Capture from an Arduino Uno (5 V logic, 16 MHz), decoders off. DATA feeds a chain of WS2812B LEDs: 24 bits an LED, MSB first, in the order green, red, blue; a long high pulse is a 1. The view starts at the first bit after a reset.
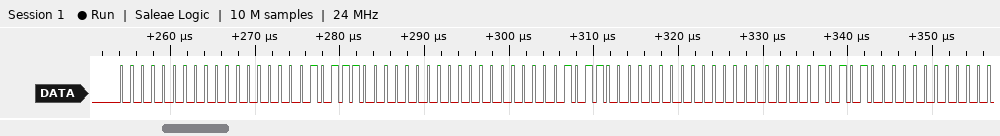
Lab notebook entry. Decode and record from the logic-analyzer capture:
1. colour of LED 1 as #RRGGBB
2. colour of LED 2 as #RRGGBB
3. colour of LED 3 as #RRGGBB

#00002E
#00002C
#00002A
